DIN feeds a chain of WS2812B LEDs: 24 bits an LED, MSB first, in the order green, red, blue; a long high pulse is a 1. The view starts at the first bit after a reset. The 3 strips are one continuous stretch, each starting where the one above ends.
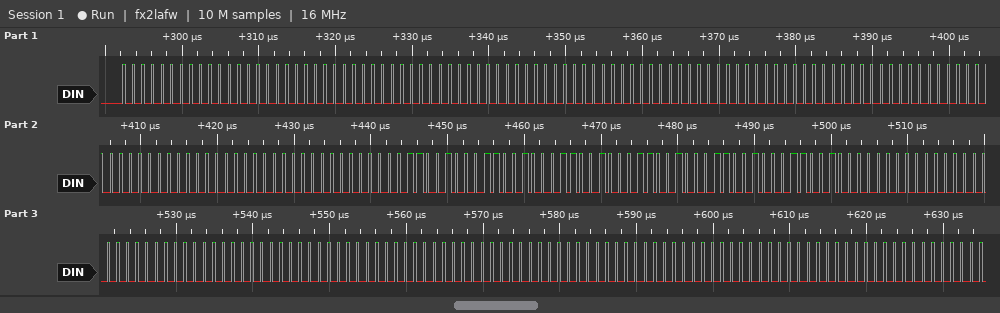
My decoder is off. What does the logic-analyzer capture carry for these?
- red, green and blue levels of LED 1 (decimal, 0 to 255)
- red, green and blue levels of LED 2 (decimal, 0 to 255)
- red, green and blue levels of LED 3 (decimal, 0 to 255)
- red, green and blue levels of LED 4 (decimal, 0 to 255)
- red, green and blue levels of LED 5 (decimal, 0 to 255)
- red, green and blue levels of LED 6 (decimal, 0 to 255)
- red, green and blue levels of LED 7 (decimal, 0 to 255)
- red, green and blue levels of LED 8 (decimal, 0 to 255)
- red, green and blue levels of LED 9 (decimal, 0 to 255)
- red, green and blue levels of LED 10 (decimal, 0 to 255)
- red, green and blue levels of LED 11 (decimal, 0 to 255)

0, 0, 0
0, 0, 0
0, 0, 0
0, 0, 0
0, 0, 0
50, 50, 50
50, 50, 50
0, 0, 0
0, 0, 0
0, 0, 0
0, 0, 0
